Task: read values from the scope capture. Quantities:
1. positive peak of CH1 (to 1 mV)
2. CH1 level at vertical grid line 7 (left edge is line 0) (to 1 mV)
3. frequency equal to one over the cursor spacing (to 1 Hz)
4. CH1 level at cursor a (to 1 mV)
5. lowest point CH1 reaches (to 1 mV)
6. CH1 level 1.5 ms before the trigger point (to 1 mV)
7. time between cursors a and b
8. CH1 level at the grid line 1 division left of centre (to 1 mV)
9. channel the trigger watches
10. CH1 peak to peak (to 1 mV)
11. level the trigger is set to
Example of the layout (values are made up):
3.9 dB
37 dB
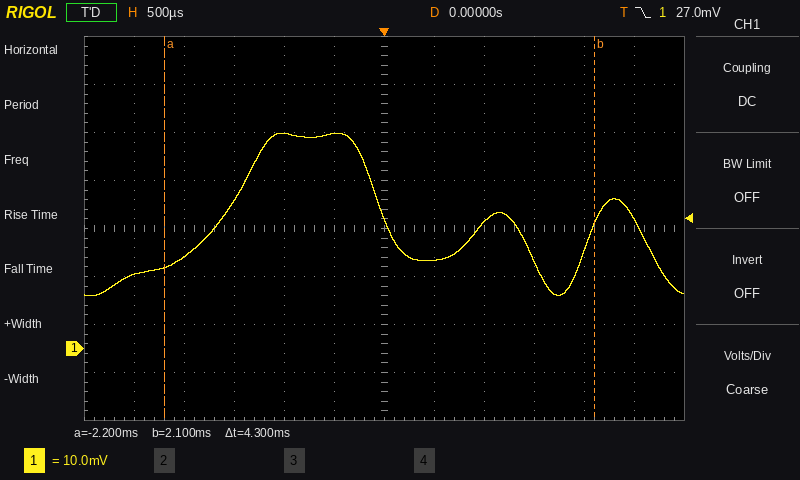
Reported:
45 mV
18 mV
233 Hz
17 mV
11 mV
31 mV
4.3 ms
45 mV
CH1
34 mV
27.0 mV
